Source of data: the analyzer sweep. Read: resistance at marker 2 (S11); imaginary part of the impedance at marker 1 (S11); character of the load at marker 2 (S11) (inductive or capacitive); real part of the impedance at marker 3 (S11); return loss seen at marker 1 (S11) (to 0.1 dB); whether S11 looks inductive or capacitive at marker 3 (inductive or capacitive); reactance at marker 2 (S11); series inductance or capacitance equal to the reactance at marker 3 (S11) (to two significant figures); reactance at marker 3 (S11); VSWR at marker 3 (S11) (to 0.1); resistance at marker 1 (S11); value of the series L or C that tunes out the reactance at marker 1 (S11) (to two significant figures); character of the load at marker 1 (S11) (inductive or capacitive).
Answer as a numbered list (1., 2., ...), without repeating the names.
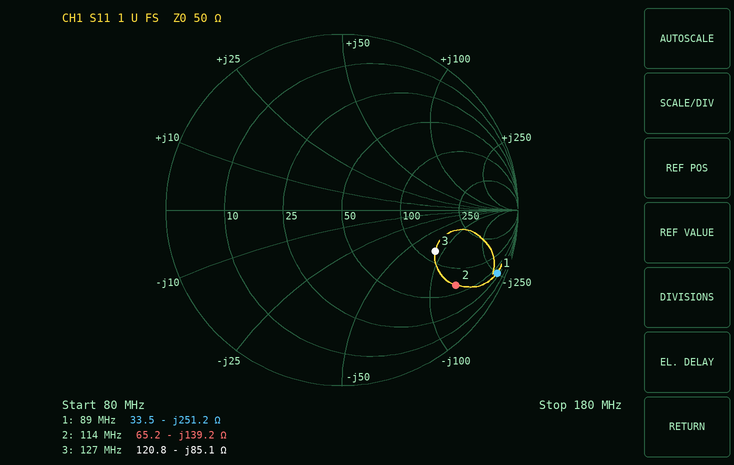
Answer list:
1. 65.2 Ω
2. -251.2 Ω
3. capacitive
4. 120.8 Ω
5. 0.4 dB
6. capacitive
7. -139.2 Ω
8. 15 pF
9. -85.1 Ω
10. 3.8
11. 33.5 Ω
12. 450 nH
13. capacitive
